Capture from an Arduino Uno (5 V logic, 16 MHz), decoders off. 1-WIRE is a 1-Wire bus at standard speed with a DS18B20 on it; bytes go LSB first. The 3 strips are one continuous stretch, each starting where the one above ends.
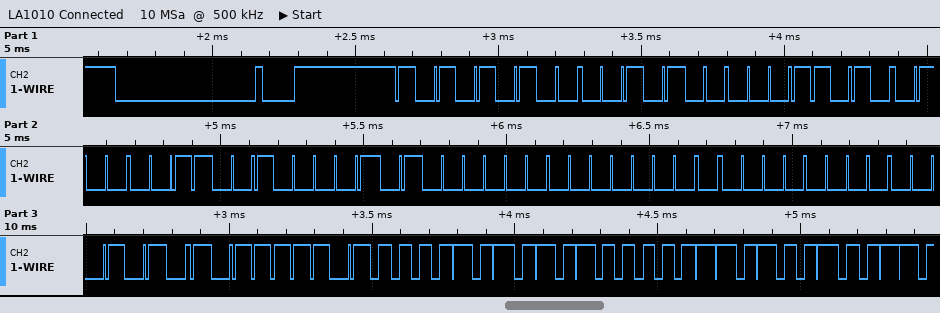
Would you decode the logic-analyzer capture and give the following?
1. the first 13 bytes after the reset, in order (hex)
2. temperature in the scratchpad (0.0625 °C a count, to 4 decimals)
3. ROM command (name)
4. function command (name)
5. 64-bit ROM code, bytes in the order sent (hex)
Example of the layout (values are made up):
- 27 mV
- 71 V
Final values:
- 55 28 58 C2 84 02 00 00 A8 BE 50 05 4B
- 85.0000 °C
- Match ROM
- Read Scratchpad
- 28 58 C2 84 02 00 00 A8
